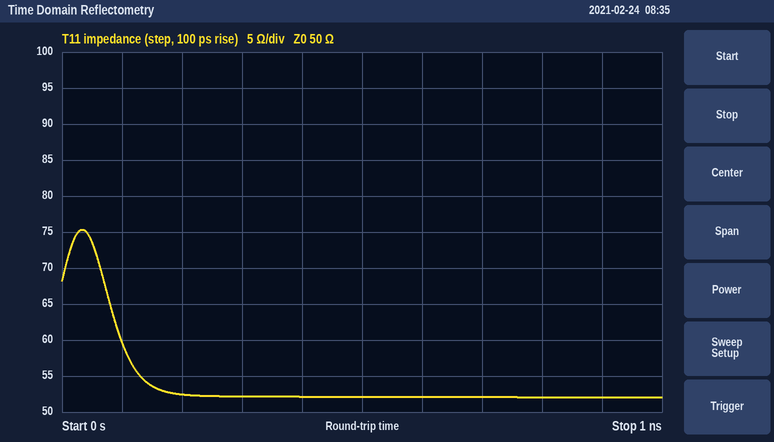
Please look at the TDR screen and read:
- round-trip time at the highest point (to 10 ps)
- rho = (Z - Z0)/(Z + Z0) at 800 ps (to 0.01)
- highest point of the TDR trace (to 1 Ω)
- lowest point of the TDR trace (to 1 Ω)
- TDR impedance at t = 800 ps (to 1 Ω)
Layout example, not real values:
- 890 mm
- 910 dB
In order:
- 30 ps
- +0.02
- 75 Ω
- 52 Ω
- 52 Ω
